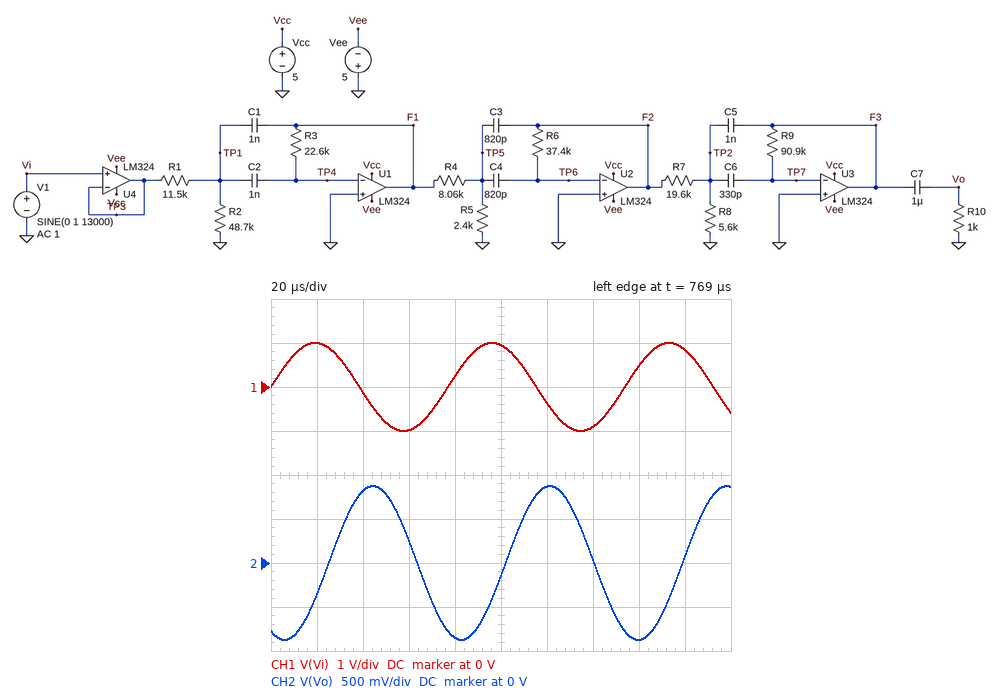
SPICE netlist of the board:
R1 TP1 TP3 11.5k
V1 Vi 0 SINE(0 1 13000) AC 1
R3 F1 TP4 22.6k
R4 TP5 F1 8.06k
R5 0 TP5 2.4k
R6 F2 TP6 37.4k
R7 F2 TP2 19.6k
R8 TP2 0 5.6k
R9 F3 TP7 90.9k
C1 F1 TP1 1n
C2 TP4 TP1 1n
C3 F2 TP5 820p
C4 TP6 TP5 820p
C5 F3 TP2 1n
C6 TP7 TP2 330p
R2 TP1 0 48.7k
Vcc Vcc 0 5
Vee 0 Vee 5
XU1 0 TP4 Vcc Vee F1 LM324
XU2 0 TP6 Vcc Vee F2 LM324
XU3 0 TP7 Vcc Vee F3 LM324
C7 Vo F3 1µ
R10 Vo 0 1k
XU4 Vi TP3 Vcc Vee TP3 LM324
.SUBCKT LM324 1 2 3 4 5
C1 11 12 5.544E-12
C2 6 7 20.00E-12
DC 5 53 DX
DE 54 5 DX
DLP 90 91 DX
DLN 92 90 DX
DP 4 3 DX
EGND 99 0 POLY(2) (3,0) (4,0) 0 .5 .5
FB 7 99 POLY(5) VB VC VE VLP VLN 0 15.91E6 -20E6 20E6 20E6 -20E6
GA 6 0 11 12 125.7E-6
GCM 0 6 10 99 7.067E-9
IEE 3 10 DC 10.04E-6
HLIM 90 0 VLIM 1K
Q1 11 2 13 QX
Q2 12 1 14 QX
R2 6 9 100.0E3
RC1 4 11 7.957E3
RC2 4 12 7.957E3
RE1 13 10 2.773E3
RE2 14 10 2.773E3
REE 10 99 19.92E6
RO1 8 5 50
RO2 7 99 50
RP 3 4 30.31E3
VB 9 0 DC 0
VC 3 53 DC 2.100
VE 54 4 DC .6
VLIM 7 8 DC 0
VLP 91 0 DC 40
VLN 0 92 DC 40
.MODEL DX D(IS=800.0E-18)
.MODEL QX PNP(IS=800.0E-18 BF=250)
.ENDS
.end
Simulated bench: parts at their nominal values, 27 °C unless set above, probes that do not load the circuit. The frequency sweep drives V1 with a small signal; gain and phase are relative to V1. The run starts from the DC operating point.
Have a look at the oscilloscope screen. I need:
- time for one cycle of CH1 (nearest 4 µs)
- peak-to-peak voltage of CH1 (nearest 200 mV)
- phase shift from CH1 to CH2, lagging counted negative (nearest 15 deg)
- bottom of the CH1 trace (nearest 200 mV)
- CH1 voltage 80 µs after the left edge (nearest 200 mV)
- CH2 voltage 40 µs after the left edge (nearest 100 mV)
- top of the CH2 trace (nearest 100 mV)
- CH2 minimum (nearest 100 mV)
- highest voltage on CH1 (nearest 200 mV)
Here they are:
76 µs
2.0 V
-120 deg
-1.0 V
200 mV
800 mV
900 mV
-900 mV
1.0 V
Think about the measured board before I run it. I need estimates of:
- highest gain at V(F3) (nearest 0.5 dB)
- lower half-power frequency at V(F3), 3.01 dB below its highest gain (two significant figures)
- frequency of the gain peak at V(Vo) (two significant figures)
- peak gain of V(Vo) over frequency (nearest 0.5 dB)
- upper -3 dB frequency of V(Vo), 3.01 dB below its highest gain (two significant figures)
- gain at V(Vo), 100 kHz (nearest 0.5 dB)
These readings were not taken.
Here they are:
0 dB
12 kHz
15 kHz
0 dB
22 kHz
-52.0 dB
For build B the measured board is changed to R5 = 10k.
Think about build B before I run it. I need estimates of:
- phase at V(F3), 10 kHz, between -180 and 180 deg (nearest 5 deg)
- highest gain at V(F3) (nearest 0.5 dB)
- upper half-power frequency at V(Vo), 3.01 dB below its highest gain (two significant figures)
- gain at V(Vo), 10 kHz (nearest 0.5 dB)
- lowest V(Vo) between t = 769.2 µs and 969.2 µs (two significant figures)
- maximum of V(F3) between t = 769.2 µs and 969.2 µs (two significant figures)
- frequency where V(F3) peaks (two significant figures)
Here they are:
-75 deg
7.5 dB
16 kHz
0.5 dB
-2.3 V
2.3 V
14 kHz
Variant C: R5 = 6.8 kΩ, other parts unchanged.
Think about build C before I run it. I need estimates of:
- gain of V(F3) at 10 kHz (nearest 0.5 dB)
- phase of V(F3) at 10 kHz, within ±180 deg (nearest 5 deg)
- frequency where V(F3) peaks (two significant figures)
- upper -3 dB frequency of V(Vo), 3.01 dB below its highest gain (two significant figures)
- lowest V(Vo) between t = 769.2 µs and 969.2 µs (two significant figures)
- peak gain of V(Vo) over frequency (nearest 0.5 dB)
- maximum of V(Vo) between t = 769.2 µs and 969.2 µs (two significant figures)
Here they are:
-1.5 dB
-65 deg
14 kHz
17 kHz
-2.0 V
7.0 dB
2.0 V
